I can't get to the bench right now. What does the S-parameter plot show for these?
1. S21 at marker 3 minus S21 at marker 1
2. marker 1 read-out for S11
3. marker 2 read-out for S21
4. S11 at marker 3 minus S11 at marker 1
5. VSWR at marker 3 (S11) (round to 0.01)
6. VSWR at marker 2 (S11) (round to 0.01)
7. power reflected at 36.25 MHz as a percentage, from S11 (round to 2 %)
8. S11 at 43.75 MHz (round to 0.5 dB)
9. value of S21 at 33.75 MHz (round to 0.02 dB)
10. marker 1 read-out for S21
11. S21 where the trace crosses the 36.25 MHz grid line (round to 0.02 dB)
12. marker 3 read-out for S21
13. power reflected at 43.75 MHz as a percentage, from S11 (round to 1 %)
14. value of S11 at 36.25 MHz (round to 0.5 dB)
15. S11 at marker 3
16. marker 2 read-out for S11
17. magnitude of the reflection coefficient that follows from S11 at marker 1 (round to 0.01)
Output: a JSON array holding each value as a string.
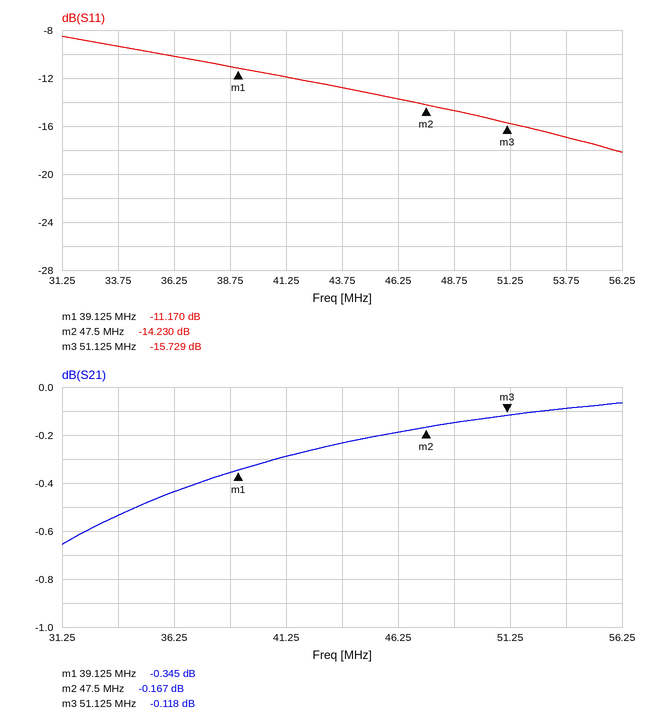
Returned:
["0.227 dB", "-11.170 dB", "-0.167 dB", "-4.559 dB", "1.39", "1.48", "10 %", "-13.0 dB", "-0.54 dB", "-0.345 dB", "-0.44 dB", "-0.118 dB", "5 %", "-10.0 dB", "-15.729 dB", "-14.230 dB", "0.28"]
